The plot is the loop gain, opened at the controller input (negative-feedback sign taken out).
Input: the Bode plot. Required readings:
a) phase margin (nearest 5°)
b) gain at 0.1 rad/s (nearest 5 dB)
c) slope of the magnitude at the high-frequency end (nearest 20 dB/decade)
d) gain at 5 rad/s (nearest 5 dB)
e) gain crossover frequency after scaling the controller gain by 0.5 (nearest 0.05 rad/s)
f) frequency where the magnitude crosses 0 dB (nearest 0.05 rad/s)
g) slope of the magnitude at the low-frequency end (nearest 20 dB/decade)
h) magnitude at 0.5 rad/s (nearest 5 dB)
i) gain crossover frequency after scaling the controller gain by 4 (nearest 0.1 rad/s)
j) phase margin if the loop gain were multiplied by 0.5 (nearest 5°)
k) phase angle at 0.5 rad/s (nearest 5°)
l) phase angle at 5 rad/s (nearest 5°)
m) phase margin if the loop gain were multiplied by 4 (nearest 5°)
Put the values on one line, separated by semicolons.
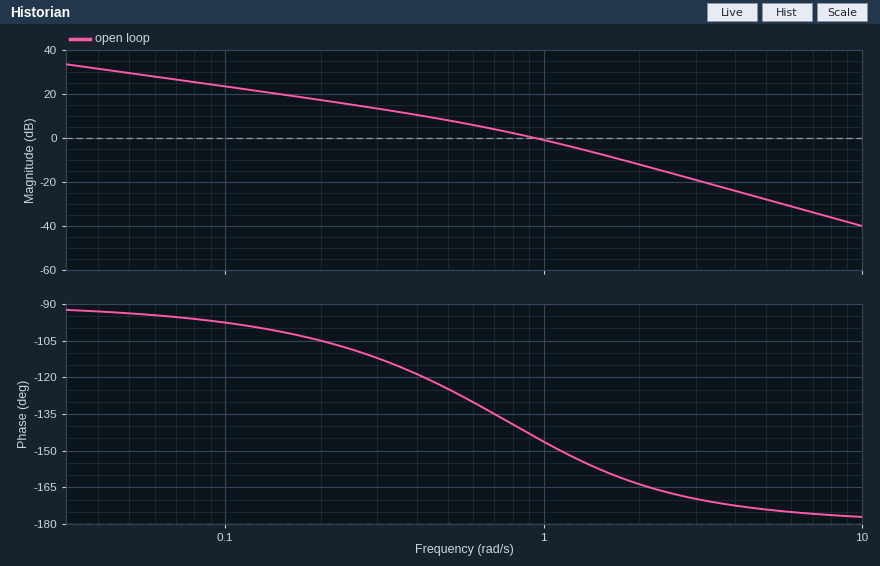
35°; 25 dB; -40 dB/decade; -30 dB; 0.60 rad/s; 0.95 rad/s; -20 dB/decade; 10 dB; 2.0 rad/s; 50°; -125°; -175°; 15°
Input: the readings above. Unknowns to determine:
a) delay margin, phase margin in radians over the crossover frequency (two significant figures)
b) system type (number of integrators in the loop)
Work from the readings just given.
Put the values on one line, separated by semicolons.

0.64 s; 1
